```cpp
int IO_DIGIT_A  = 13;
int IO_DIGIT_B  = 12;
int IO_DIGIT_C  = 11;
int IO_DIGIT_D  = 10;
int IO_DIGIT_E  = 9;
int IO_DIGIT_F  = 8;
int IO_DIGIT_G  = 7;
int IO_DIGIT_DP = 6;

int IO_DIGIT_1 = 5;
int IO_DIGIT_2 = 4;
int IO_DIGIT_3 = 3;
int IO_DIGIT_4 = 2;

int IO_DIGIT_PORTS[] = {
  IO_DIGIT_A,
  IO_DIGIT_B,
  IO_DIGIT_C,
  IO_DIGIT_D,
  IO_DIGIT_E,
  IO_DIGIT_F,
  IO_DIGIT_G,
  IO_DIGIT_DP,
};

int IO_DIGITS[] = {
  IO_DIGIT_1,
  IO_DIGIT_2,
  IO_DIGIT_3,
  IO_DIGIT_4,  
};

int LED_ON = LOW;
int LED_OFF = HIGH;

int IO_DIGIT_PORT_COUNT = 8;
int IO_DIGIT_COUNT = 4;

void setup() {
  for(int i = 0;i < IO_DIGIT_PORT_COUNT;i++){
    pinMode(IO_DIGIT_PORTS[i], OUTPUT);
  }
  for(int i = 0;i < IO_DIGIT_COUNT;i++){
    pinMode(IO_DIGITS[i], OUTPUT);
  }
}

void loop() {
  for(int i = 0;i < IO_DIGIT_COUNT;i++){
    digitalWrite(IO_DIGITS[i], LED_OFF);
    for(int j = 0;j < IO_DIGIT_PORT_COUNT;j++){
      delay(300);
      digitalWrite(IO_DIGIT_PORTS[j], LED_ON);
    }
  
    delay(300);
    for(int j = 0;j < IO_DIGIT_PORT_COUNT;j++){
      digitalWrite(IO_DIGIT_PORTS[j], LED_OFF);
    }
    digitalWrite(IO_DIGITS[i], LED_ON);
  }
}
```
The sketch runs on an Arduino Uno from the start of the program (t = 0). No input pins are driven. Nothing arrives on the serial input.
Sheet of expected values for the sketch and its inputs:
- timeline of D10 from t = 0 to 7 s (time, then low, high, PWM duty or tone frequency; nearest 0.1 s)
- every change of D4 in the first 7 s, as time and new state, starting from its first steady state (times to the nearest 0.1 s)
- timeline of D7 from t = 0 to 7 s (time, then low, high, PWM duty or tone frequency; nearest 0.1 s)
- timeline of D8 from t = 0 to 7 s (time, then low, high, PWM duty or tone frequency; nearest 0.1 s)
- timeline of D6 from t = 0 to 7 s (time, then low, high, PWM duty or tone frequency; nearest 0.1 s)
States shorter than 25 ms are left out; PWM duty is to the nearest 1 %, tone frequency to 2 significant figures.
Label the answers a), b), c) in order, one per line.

a) 0 s low; 2.7 s high; 3.9 s low; 5.4 s high; 6.6 s low
b) 0 s low; 2.7 s high; 5.4 s low
c) 0 s low; 2.7 s high; 4.8 s low; 5.4 s high
d) 0 s low; 2.7 s high; 4.5 s low; 5.4 s high
e) 0 s low; 2.7 s high; 5.1 s low; 5.4 s high
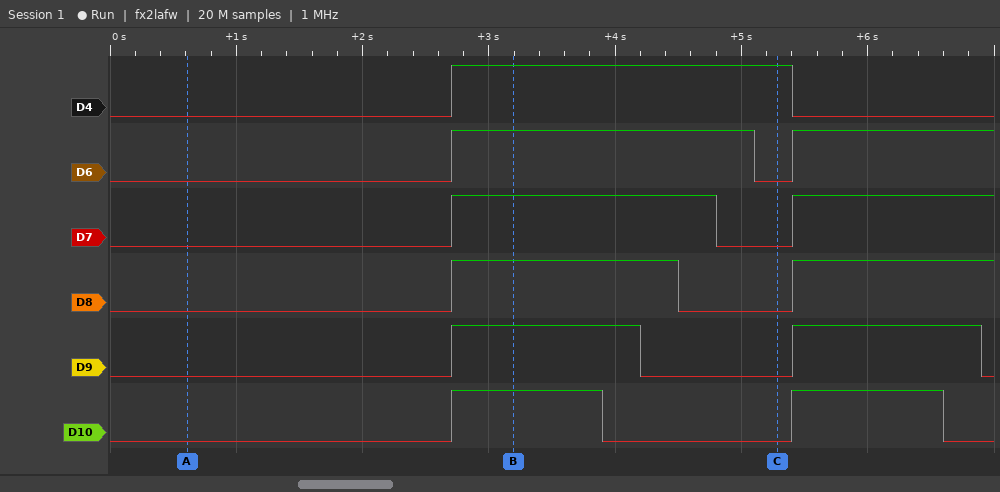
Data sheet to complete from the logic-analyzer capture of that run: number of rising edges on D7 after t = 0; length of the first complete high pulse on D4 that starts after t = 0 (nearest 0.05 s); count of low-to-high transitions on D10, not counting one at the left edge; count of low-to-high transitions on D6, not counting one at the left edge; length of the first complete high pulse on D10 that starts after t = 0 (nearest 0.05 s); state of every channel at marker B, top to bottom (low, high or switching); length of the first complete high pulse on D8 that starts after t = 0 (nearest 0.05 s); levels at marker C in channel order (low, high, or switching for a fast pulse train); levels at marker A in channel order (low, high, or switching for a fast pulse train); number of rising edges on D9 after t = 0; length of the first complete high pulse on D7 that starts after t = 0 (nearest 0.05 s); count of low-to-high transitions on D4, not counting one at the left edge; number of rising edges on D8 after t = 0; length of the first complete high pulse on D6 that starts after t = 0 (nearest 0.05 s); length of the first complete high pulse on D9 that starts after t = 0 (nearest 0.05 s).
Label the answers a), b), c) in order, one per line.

a) 2
b) 2.70 s
c) 2
d) 2
e) 1.20 s
f) D4 high, D6 high, D7 high, D8 high, D9 high, D10 high
g) 1.80 s
h) D4 high, D6 low, D7 low, D8 low, D9 low, D10 low
i) D4 low, D6 low, D7 low, D8 low, D9 low, D10 low
j) 2
k) 2.10 s
l) 1
m) 2
n) 2.40 s
o) 1.50 s
